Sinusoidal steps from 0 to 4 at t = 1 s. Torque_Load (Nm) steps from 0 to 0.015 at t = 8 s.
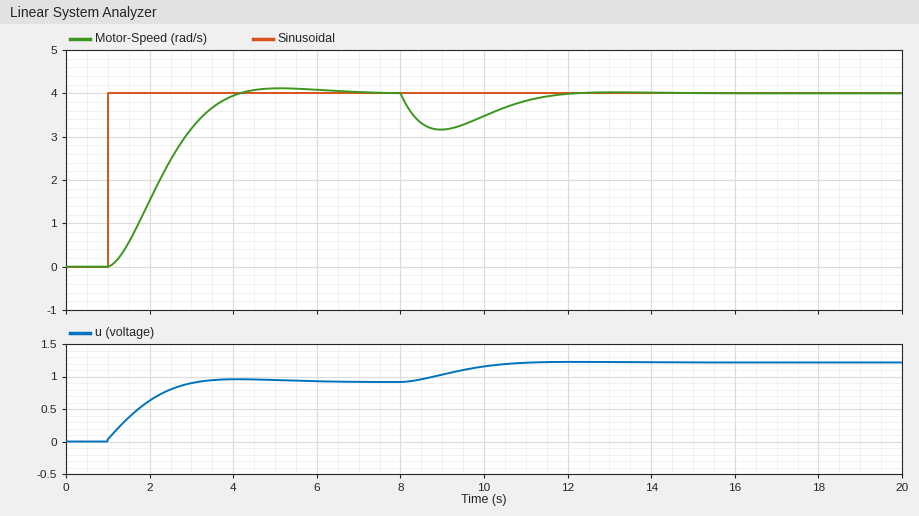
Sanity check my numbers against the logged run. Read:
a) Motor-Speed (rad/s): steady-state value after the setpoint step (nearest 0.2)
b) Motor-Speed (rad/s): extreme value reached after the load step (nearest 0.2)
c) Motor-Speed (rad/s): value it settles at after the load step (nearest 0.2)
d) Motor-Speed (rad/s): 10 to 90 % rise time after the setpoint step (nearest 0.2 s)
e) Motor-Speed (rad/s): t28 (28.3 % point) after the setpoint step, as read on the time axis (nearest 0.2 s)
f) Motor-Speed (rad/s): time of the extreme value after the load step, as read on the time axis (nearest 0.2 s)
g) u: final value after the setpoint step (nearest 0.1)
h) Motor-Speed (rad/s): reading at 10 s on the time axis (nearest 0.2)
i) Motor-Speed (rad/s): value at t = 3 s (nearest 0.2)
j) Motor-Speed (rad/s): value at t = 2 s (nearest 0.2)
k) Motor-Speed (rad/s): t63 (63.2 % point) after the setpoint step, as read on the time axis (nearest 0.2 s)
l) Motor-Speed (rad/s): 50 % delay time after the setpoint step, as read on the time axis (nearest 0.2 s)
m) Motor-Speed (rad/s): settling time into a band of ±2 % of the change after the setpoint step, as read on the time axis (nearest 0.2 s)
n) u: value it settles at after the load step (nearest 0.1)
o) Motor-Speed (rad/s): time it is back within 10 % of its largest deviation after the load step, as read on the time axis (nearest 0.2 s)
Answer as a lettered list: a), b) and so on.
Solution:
a) 4.0
b) 3.2
c) 4.0
d) 2.0 s
e) 1.8 s
f) 9.0 s
g) 0.9
h) 3.4
i) 3.2
j) 1.6
k) 2.6 s
l) 2.2 s
m) 6.0 s
n) 1.2
o) 11.4 s
